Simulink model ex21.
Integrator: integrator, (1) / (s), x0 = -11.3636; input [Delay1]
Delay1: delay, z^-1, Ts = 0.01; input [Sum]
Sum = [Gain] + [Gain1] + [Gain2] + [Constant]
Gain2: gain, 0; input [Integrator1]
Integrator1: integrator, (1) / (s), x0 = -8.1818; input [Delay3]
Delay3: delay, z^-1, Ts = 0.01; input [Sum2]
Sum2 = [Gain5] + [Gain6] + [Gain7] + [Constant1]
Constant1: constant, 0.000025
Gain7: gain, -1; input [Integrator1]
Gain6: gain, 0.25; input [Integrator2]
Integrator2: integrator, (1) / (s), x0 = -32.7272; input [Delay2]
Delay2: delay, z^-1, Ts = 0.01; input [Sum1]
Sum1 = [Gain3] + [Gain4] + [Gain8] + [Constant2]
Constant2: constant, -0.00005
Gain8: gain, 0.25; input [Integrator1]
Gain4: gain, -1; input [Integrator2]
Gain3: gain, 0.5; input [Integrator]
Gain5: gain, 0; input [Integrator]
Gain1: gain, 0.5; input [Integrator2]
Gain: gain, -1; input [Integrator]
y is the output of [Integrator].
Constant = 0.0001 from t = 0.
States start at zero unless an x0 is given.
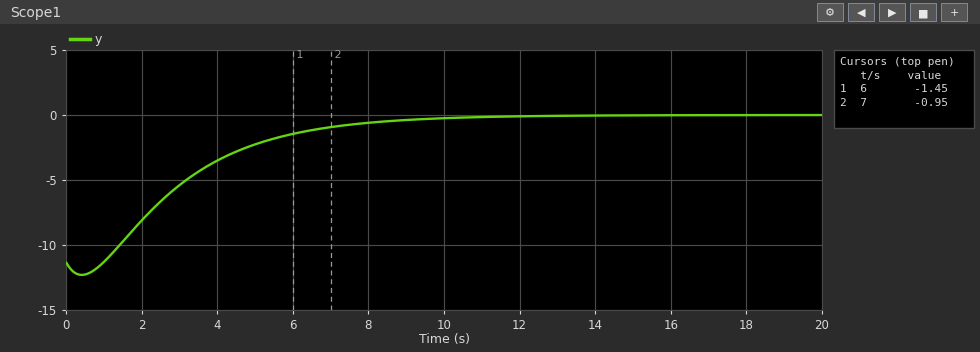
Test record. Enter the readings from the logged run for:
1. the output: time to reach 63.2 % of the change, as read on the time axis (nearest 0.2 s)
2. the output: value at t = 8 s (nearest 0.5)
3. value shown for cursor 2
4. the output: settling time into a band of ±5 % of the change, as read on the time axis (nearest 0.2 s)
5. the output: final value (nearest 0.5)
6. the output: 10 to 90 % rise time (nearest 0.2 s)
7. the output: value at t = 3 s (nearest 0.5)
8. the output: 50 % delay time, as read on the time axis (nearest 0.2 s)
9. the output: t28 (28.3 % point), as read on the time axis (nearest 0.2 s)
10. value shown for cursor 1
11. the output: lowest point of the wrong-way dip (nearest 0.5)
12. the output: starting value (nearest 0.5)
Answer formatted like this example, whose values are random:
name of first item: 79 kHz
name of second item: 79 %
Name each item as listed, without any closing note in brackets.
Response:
the output: time to reach 63.2 % of the change, as read on the time axis: 3.6 s
the output: value at t = 8 s: -0.5
value shown for cursor 2: -0.95
the output: settling time into a band of ±5 % of the change, as read on the time axis: 8.2 s
the output: final value: 0.0
the output: 10 to 90 % rise time: 5.2 s
the output: value at t = 3 s: -5.5
the output: 50 % delay time, as read on the time axis: 2.8 s
the output: t28 (28.3 % point), as read on the time axis: 2.0 s
value shown for cursor 1: -1.45
the output: lowest point of the wrong-way dip: -12.5
the output: starting value: -11.5
